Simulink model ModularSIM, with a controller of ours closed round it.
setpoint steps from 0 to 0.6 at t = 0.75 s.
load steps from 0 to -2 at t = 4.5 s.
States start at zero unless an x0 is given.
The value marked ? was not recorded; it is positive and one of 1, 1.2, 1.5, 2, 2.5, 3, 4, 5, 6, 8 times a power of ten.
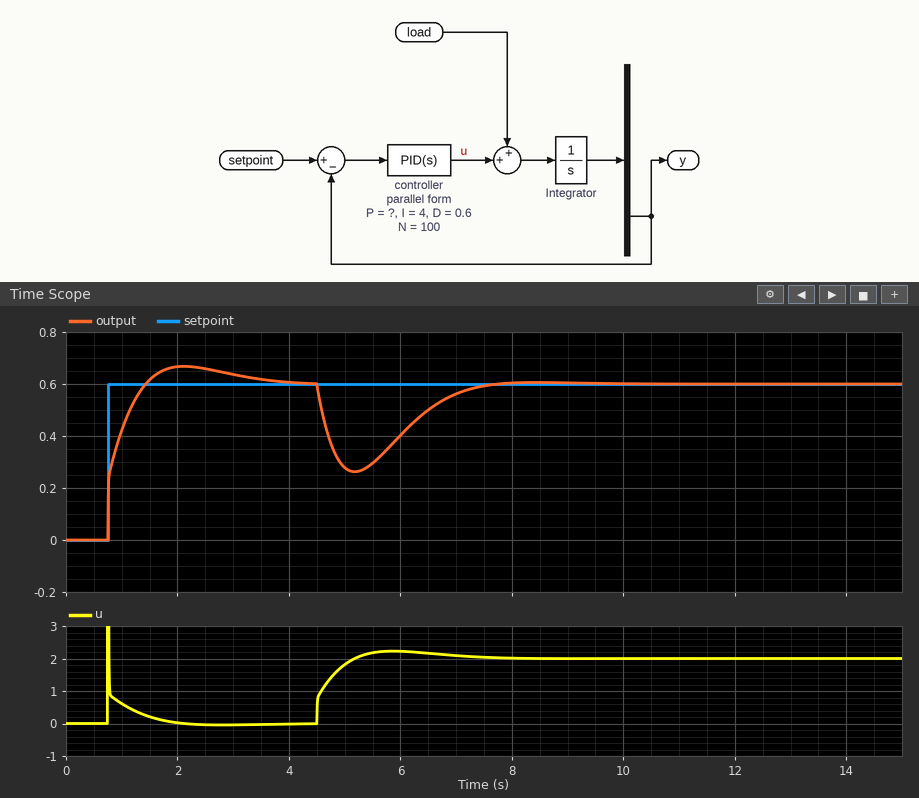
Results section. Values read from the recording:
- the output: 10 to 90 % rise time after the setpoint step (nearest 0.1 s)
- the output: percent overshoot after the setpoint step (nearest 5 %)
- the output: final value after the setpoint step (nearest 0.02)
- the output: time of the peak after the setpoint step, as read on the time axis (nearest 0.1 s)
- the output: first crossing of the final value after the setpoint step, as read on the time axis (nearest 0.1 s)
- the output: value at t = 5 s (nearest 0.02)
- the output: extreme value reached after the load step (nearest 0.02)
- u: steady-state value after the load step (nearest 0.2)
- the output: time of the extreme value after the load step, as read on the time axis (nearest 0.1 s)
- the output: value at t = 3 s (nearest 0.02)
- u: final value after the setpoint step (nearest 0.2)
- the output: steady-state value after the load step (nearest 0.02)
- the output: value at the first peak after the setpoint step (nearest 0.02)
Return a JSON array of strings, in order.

["0.5 s", "10 %", "0.60", "2.1 s", "1.4 s", "0.28", "0.26", "2.0", "5.2 s", "0.64", "0.0", "0.60", "0.66"]
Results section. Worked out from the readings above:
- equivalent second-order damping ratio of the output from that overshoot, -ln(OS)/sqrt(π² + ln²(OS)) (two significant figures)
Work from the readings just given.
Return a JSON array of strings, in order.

["0.59"]
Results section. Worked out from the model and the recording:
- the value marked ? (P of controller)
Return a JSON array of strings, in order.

["4"]
